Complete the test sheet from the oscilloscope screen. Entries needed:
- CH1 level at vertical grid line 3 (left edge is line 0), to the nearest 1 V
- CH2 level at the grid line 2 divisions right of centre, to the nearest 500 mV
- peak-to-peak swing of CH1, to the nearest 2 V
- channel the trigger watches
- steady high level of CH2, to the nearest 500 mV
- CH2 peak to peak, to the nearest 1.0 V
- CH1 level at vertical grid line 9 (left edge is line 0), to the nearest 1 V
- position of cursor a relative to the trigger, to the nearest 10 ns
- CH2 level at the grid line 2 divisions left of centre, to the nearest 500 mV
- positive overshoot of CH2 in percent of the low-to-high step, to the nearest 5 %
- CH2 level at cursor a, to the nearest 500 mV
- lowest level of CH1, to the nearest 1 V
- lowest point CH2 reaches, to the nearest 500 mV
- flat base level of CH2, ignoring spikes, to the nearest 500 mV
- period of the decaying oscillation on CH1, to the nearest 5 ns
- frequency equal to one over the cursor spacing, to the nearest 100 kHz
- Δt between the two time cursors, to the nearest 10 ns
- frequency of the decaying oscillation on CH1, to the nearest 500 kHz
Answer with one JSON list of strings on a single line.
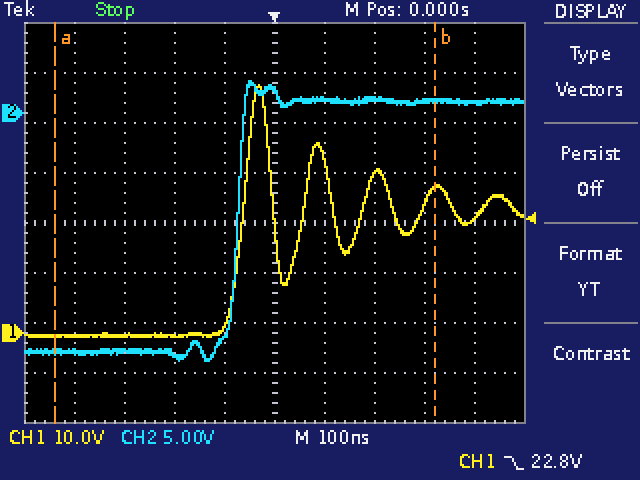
["-1 V", "1.5 V", "50 V", "CH1", "1.0 V", "28.0 V", "23 V", "-440 ns", "-24.0 V", "10 %", "-24.0 V", "-1 V", "-25.0 V", "-24.0 V", "120 ns", "1.3 MHz", "760 ns", "8.5 MHz"]
